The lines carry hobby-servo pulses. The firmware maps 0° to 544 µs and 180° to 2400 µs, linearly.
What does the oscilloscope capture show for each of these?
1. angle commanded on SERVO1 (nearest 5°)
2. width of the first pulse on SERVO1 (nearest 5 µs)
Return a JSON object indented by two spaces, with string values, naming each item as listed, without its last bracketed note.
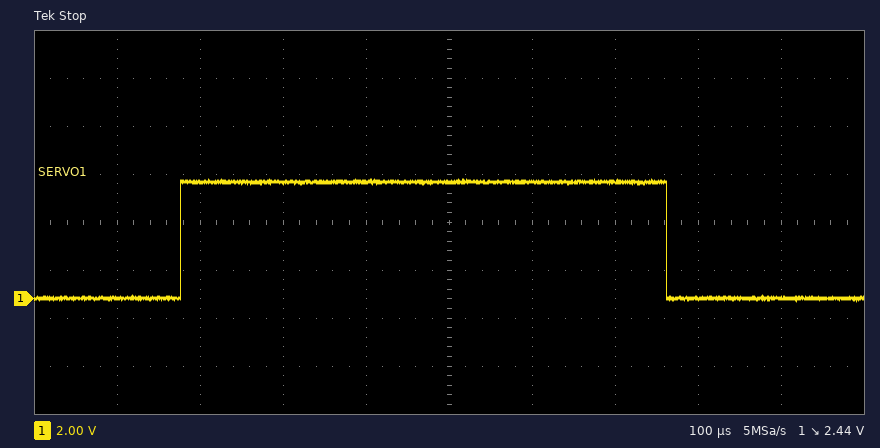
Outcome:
{
  "angle commanded on SERVO1": "5°",
  "width of the first pulse on SERVO1": "585 µs"
}
